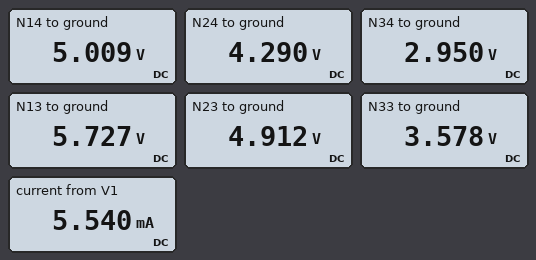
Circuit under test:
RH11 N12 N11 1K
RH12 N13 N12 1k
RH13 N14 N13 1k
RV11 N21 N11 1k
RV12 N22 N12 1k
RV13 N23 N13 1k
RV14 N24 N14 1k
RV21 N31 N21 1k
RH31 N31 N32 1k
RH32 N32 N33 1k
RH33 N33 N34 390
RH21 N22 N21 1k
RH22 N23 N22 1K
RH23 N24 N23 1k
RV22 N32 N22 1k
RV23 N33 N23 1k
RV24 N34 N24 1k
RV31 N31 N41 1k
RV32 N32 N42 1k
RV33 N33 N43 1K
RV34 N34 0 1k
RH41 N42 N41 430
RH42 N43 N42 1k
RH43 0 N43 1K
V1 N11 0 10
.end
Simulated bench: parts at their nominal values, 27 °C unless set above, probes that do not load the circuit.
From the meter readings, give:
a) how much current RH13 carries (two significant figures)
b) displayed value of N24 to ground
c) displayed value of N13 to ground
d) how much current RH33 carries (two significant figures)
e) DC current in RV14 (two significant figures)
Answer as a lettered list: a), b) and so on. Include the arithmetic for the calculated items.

a) (5.727 V - 5.009 V) / 1 kΩ = 720 µA
b) 4.290 V
c) 5.727 V
d) (3.578 V - 2.95 V) / 390 Ω = 1.6 mA
e) (5.009 V - 4.29 V) / 1 kΩ = 720 µA
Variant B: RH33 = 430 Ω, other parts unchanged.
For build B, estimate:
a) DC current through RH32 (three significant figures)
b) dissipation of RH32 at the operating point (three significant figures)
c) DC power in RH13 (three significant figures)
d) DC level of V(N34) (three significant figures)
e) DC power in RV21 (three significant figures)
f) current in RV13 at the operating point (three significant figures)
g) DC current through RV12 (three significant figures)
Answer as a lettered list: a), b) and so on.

a) 1.25 mA
b) 1.57 mW
c) 522 µW
d) 2.93 V
e) 2.72 mW
f) 811 µA
g) 1.20 mA
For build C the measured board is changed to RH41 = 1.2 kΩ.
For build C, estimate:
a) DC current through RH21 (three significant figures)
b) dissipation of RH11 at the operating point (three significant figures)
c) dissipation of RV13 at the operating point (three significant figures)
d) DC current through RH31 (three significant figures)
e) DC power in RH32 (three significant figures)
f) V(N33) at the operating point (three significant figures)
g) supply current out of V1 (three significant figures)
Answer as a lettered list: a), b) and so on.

a) 1.18 mA
b) 7.48 mW
c) 666 µW
d) 835 µA
e) 1.63 mW
f) 3.57 V
g) 5.49 mA
